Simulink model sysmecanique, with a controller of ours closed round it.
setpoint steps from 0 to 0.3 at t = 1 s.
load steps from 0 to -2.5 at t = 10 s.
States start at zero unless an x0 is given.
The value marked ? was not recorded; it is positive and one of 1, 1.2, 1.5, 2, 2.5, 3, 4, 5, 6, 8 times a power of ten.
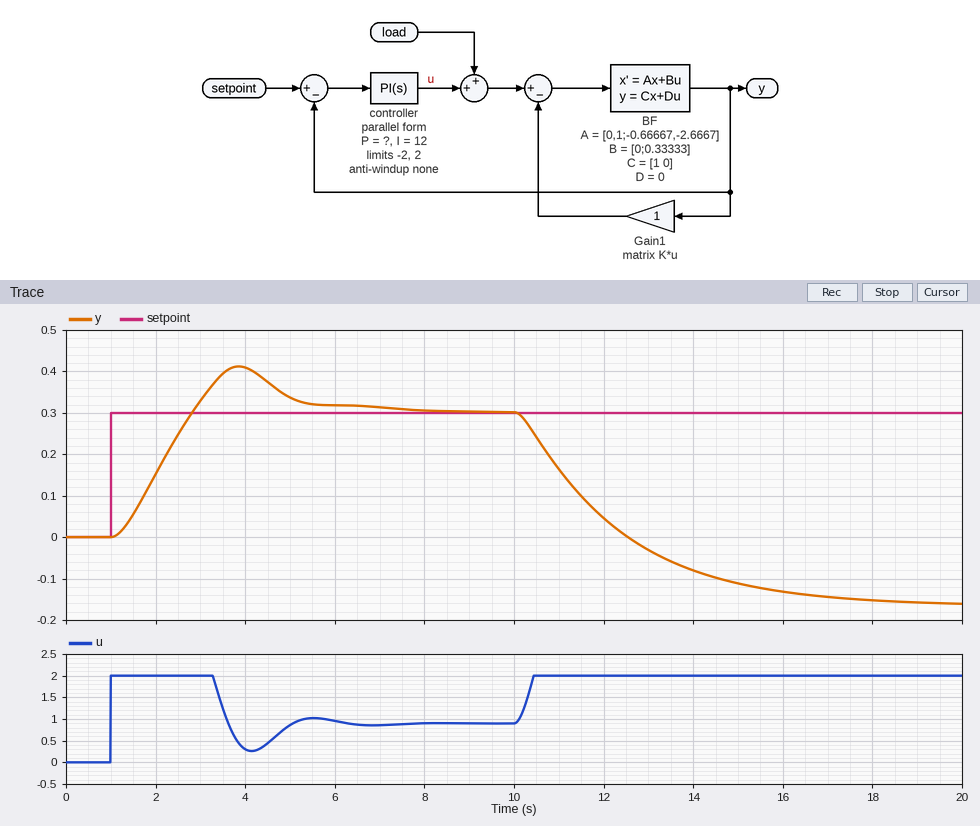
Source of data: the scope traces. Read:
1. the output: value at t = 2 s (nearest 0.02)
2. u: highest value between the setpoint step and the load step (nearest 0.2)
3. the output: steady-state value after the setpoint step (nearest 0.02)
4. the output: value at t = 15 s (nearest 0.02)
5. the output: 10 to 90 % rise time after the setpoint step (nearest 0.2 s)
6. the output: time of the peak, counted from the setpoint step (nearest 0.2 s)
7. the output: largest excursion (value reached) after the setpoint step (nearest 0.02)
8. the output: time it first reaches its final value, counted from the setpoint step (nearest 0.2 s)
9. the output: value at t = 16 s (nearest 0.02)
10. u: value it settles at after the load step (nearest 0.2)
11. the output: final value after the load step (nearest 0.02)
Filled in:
0.16
2.0
0.30
-0.12
1.2 s
2.8 s
0.42
1.8 s
-0.14
2.0
-0.16
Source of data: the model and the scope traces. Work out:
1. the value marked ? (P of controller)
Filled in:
20
